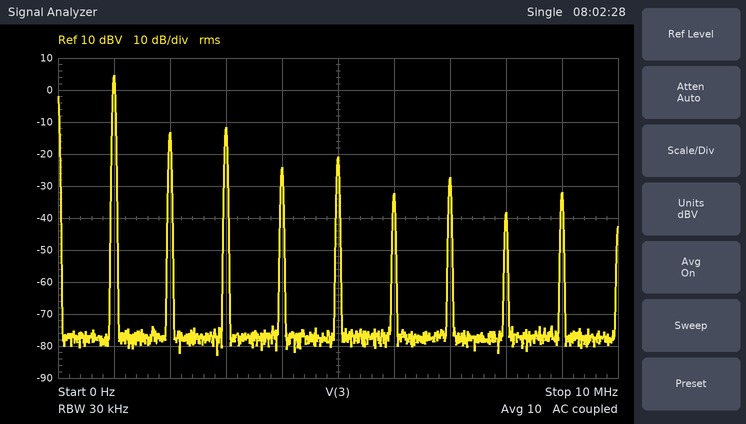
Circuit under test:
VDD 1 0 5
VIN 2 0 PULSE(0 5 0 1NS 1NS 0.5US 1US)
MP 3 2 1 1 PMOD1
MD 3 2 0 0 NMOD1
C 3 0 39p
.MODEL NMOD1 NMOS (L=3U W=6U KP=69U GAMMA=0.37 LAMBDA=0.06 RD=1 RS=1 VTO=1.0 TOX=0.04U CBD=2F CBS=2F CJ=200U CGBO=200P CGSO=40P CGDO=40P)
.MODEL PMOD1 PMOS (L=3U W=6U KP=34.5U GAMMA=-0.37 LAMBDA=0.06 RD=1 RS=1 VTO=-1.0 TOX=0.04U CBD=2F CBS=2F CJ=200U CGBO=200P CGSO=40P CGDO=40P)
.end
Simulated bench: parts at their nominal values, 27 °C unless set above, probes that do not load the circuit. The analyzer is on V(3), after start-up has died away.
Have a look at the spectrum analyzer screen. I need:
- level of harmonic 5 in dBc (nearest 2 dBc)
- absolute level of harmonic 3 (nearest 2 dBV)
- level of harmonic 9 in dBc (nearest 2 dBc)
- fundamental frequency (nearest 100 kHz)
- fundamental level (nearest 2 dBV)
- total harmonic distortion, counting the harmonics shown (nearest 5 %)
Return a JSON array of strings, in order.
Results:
["-26 dBc", "-12 dBV", "-36 dBc", "1.0 MHz", "4 dBV", "20 %"]
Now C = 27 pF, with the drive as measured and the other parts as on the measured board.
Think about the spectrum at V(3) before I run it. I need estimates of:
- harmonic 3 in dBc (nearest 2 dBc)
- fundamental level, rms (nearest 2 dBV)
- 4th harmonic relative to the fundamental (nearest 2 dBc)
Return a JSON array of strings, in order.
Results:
["-14 dBc", "6 dBV", "-26 dBc"]
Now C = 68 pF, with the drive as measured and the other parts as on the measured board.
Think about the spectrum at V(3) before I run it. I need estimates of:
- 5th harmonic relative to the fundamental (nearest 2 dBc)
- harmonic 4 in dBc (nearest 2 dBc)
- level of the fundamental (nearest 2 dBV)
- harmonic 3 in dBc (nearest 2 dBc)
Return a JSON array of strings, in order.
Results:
["-28 dBc", "-32 dBc", "2 dBV", "-18 dBc"]
